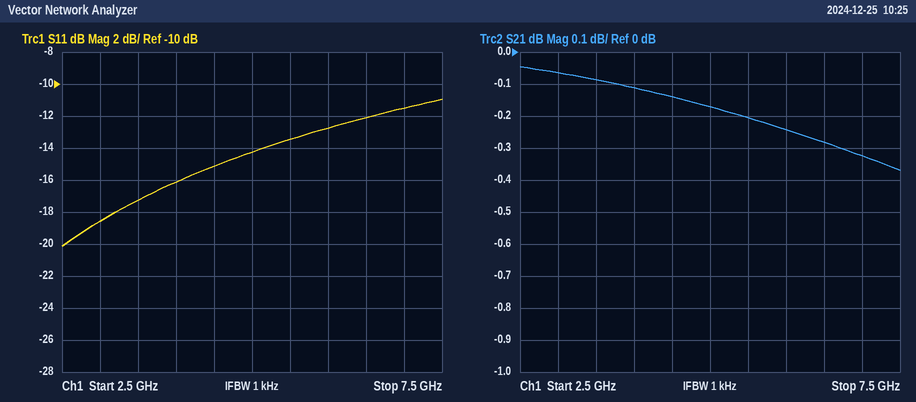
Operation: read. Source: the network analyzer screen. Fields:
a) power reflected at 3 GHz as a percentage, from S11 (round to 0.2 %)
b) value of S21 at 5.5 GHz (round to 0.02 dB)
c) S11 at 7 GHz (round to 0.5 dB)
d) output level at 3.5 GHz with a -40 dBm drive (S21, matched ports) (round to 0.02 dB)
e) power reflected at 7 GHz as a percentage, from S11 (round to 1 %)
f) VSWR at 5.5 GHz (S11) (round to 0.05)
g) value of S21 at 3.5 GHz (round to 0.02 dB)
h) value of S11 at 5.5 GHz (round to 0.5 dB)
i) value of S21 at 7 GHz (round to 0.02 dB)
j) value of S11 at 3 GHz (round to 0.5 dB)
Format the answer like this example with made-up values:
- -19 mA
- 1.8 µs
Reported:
- 1.4 %
- -0.20 dB
- -11.5 dB
- -40.08 dBm
- 7 %
- 1.55
- -0.08 dB
- -13.5 dB
- -0.32 dB
- -18.5 dB
